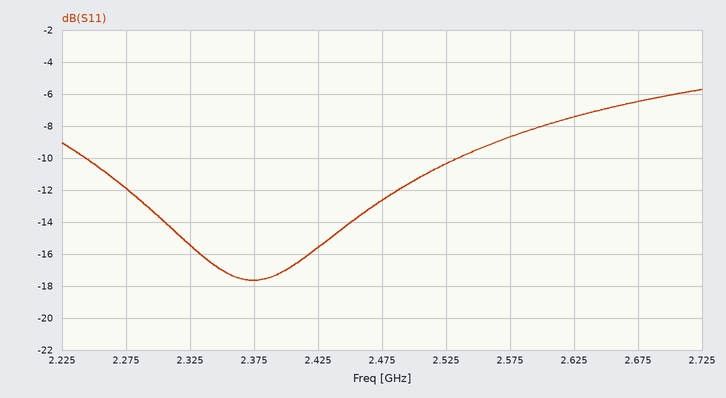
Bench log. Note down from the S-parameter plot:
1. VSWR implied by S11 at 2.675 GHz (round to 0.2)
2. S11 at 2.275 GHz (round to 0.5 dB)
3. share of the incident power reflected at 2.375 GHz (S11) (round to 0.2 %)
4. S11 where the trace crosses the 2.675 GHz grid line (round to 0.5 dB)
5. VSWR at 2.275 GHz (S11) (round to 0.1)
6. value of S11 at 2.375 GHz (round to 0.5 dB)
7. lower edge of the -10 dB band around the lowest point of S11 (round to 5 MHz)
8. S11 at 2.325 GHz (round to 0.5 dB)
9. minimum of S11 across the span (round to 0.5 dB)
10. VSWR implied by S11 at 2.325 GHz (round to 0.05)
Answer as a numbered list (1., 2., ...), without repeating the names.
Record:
1. 2.8
2. -12.0 dB
3. 1.8 %
4. -6.5 dB
5. 1.7
6. -17.5 dB
7. 2.245 GHz
8. -15.5 dB
9. -17.5 dB
10. 1.40
